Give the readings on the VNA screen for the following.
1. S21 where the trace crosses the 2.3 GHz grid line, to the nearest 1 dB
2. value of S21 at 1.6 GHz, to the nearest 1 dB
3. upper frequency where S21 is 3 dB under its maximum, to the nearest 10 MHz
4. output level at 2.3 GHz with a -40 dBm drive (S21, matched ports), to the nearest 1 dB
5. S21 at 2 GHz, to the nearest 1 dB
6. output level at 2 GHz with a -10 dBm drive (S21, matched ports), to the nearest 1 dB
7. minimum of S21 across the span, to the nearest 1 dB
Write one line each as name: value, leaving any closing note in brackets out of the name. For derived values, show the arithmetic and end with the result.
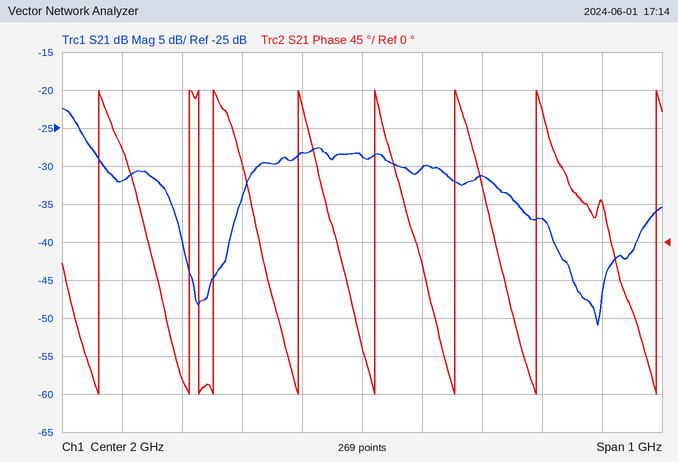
S21 where the trace crosses the 2.3 GHz grid line, to the nearest 1 dB: -37 dB
value of S21 at 1.6 GHz, to the nearest 1 dB: -32 dB
upper frequency where S21 is 3 dB under its maximum, to the nearest 10 MHz: 1.53 GHz
output level at 2.3 GHz with a -40 dBm drive (S21, matched ports), to the nearest 1 dB: -40 dBm + (-37 dB) = -77 dBm
S21 at 2 GHz, to the nearest 1 dB: -29 dB
output level at 2 GHz with a -10 dBm drive (S21, matched ports), to the nearest 1 dB: -10 dBm + (-29 dB) = -39 dBm
minimum of S21 across the span, to the nearest 1 dB: -51 dB
